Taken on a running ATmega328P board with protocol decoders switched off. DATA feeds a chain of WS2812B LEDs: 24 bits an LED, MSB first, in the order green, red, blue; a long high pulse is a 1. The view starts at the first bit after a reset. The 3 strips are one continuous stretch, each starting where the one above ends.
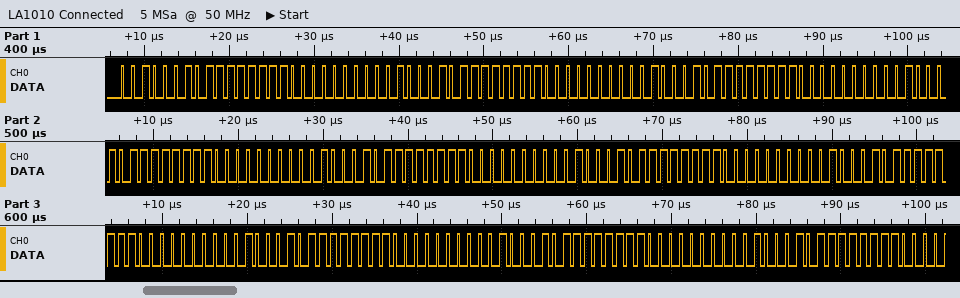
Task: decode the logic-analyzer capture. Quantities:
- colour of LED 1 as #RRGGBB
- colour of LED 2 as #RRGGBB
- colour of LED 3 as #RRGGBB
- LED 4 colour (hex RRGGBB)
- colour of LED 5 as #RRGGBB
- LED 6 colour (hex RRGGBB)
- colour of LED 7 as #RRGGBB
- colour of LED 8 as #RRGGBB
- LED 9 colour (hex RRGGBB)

#FF2200
#FF2200
#FF2200
#FF2200
#FF2200
#FF2200
#FF2200
#FF2200
#FF2200
